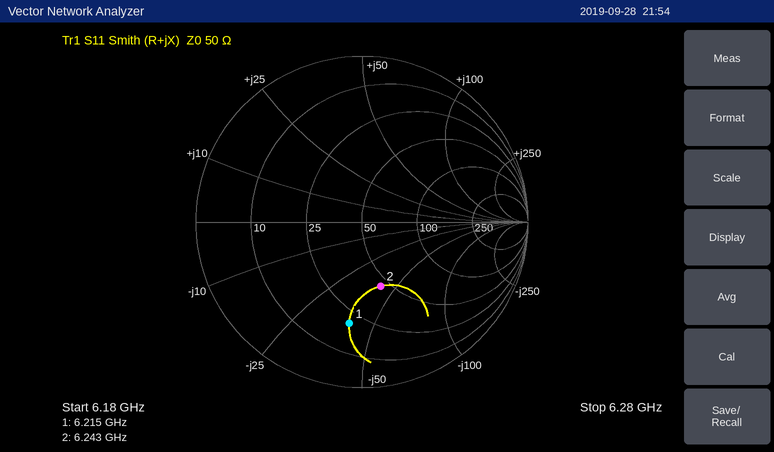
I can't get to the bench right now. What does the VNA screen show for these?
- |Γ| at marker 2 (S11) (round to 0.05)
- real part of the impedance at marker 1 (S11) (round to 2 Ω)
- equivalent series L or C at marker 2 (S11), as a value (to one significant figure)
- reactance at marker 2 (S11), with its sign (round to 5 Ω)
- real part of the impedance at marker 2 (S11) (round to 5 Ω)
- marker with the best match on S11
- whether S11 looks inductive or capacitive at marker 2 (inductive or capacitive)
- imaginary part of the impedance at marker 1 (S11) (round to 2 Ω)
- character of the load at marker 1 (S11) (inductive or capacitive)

0.40
20 Ω
600 fF
-40 Ω
45 Ω
marker 2
capacitive
-40 Ω
capacitive
